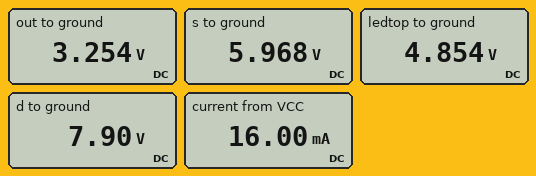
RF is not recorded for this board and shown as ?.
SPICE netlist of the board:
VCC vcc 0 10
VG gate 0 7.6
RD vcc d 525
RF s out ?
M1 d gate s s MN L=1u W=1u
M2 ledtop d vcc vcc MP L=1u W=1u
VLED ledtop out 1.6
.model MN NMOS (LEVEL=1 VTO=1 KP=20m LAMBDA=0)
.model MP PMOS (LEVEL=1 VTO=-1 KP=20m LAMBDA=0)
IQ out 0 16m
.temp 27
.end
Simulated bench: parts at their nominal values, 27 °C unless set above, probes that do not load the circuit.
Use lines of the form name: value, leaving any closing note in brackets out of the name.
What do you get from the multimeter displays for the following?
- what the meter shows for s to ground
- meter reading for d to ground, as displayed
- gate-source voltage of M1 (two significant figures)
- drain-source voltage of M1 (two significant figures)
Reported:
what the meter shows for s to ground: 5.968 V
meter reading for d to ground, as displayed: 7.90 V
gate-source voltage of M1: 1.6 V
drain-source voltage of M1: 1.9 V
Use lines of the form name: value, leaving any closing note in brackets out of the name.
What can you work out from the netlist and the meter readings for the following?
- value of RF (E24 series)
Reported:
value of RF: 680 Ω
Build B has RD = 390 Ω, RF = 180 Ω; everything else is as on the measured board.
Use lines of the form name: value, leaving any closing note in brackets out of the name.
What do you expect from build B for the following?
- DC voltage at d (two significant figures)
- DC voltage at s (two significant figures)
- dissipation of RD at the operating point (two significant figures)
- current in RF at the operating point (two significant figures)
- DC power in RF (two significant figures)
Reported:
DC voltage at d: 8.0 V
DC voltage at s: 5.9 V
dissipation of RD at the operating point: 11 mW
current in RF at the operating point: 5.2 mA
DC power in RF: 4.9 mW
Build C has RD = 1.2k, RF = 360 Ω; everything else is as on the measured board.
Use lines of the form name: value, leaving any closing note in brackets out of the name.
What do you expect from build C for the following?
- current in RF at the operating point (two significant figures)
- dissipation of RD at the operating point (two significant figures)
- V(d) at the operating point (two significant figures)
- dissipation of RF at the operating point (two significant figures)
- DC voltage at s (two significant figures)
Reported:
current in RF at the operating point: 1.8 mA
dissipation of RD at the operating point: 4.0 mW
V(d) at the operating point: 7.8 V
dissipation of RF at the operating point: 1.2 mW
DC voltage at s: 6.2 V
